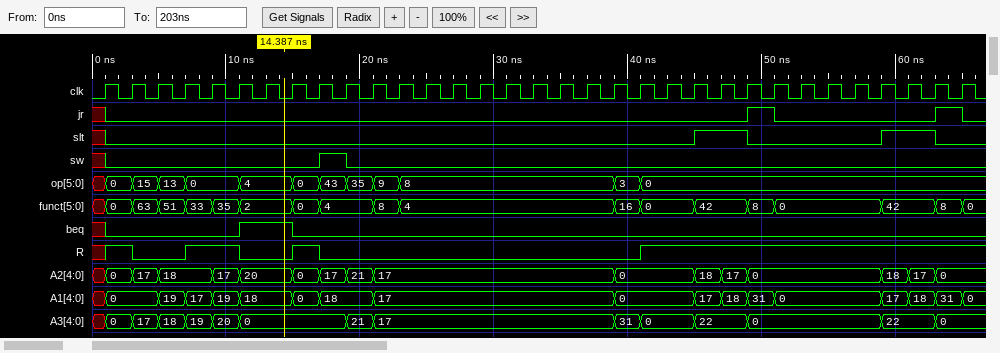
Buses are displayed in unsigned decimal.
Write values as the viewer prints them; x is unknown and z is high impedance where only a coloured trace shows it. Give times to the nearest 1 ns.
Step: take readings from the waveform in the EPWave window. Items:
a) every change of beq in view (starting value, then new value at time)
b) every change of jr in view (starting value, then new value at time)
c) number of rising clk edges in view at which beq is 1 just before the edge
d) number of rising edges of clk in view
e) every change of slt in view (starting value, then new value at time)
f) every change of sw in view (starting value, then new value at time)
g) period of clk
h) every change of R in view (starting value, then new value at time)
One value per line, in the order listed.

x, 0 at 1 ns, 1 at 11 ns, 0 at 15 ns
x, 0 at 1 ns, 1 at 49 ns, 0 at 51 ns, 1 at 63 ns, 0 at 65 ns
2
33
x, 0 at 1 ns, 1 at 45 ns, 0 at 49 ns, 1 at 59 ns, 0 at 63 ns
x, 0 at 1 ns, 1 at 17 ns, 0 at 19 ns
2 ns
x, 1 at 1 ns, 0 at 3 ns, 1 at 7 ns, 0 at 11 ns, 1 at 15 ns, 0 at 17 ns, 1 at 41 ns
